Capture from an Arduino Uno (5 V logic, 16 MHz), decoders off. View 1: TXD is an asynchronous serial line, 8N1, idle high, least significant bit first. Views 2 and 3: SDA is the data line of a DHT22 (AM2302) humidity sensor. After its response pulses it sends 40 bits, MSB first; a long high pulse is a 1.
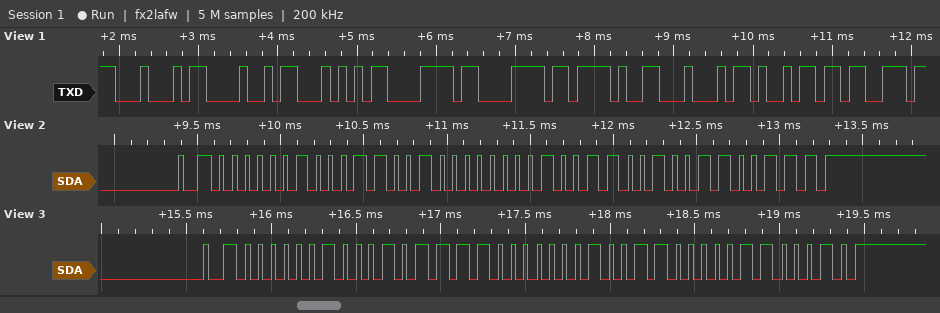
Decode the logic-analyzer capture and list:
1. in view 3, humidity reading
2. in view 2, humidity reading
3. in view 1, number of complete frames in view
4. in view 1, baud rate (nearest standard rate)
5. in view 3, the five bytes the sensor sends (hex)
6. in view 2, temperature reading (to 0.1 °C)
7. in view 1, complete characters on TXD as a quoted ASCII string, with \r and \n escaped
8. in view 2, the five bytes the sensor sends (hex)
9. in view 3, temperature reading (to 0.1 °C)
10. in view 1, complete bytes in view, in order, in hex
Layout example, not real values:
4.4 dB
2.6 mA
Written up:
55.9 %
56.2 %
9
9600 baud
02 2F 01 30 62
30.6 °C
"DHTxx/Dis"
02 32 01 32 67
30.4 °C
44 48 54 78 78 2F 44 69 73
